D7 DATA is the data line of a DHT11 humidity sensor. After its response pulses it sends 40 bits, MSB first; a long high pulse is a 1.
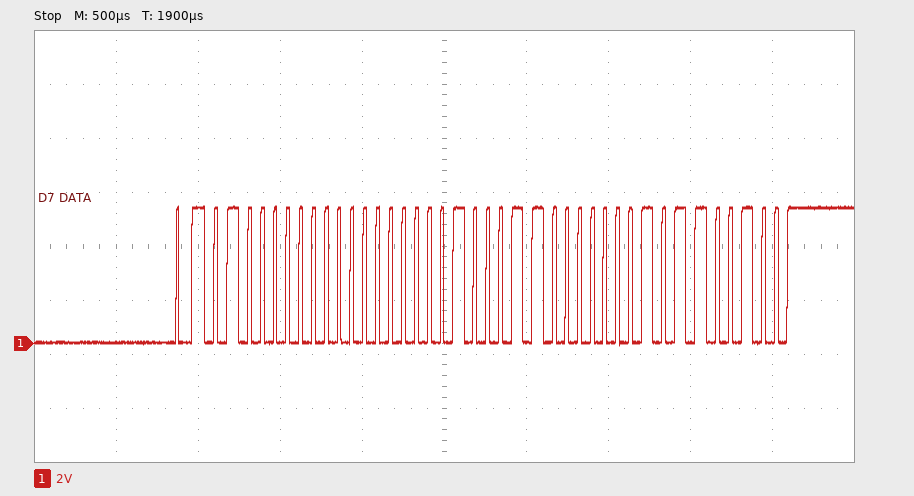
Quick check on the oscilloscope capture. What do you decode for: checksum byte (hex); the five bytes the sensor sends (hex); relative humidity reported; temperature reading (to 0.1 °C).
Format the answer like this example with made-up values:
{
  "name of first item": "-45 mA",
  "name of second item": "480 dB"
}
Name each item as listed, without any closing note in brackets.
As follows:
{
  "checksum byte": "0x64",
  "the five bytes the sensor sends": "40 00 23 01 64",
  "relative humidity reported": "64 %",
  "temperature reading": "35.1 °C"
}
